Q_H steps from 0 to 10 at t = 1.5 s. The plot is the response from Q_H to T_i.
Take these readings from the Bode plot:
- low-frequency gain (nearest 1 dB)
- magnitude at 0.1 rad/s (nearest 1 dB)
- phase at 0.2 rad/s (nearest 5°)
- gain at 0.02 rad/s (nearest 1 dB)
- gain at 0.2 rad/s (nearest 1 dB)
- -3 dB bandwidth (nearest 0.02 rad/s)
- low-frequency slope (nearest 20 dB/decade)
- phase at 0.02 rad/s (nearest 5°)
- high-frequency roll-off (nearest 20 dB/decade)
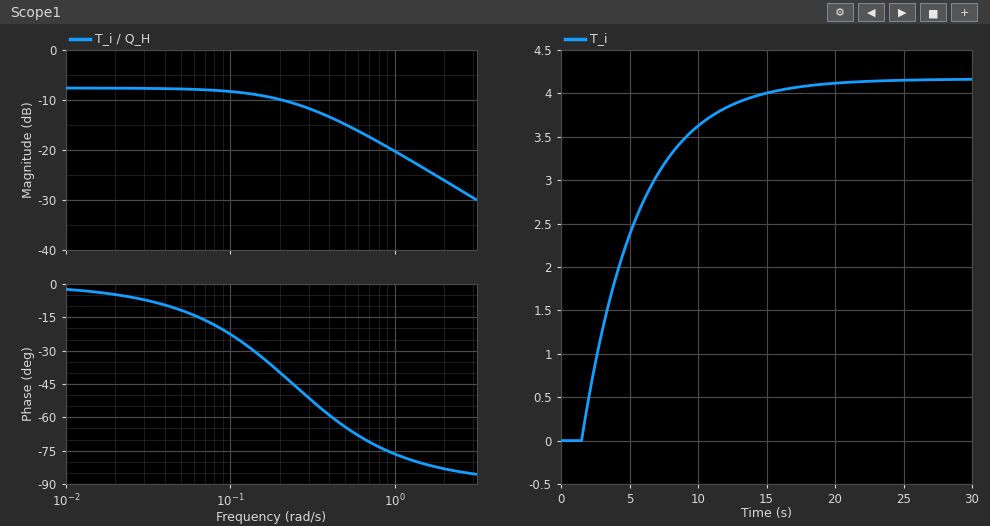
-8 dB
-8 dB
-40°
-8 dB
-10 dB
0.24 rad/s
0 dB/decade
-5°
-20 dB/decade
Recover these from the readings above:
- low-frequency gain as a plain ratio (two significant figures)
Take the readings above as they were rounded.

0.40
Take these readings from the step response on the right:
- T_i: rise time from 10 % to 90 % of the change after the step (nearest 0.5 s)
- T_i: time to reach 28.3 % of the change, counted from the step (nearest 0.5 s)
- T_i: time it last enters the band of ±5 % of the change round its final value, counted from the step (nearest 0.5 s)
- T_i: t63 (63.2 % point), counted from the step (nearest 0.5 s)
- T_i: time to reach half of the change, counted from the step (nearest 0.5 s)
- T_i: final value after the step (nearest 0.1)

9.0 s
1.5 s
12.5 s
4.0 s
3.0 s
4.2
